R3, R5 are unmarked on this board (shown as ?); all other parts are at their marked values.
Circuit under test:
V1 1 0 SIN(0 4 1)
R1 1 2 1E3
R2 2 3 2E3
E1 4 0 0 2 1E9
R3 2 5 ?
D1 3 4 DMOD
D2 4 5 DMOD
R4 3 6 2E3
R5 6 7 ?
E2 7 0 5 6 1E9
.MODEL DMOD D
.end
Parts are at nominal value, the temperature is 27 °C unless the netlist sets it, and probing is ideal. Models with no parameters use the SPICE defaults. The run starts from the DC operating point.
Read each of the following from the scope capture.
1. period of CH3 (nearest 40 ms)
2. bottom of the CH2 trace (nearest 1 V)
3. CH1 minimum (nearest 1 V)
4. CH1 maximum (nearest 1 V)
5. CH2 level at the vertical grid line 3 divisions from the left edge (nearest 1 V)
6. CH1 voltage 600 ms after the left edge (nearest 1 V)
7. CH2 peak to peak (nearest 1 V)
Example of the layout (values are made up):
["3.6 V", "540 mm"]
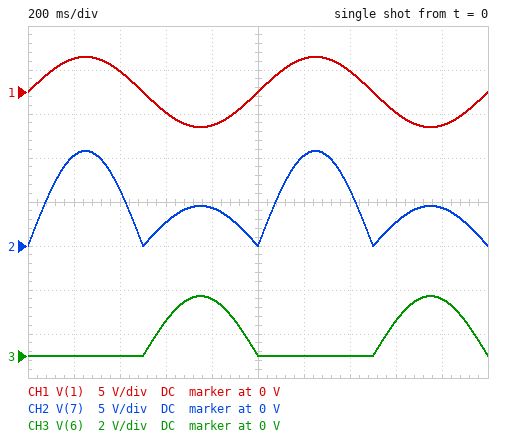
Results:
["1.00 s", "0 V", "-4 V", "4 V", "3 V", "-2 V", "11 V"]
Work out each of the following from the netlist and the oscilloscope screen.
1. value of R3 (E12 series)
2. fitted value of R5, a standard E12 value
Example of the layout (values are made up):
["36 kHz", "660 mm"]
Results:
["820 Ω", "2.7 kΩ"]
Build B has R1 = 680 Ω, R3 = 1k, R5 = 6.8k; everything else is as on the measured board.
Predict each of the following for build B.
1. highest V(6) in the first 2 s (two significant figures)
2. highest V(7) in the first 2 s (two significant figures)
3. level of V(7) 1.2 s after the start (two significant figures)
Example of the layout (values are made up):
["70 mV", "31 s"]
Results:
["4.7 V", "40 V", "38 V"]
